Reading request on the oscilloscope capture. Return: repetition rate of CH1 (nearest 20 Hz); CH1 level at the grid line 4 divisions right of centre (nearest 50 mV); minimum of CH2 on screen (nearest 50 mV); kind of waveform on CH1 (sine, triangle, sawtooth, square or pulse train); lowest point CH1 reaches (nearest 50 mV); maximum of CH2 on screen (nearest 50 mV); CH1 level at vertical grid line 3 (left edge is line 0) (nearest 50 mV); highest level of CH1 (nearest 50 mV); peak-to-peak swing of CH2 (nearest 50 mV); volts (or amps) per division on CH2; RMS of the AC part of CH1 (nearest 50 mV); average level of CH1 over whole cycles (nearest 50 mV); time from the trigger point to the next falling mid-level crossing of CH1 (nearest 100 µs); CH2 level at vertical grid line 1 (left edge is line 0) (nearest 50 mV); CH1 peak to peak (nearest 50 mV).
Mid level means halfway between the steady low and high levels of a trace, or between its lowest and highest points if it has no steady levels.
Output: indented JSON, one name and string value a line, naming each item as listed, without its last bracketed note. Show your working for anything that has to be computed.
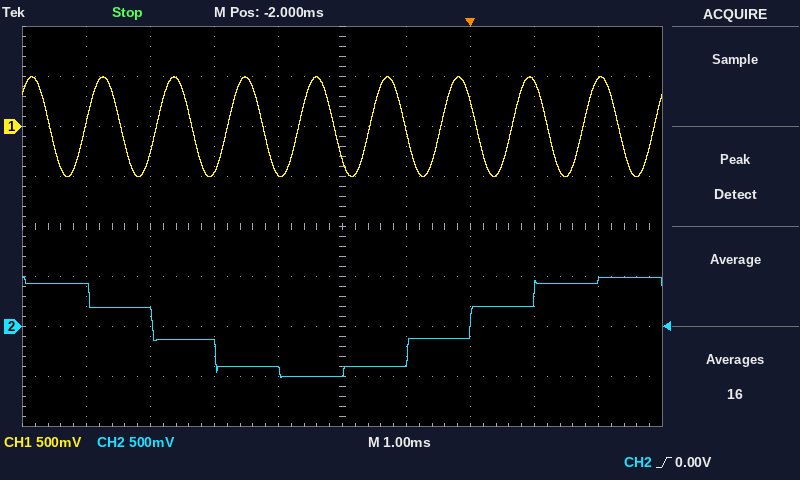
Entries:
{
  "repetition rate of CH1": "900 Hz",
  "CH1 level at the grid line 4 divisions right of centre": "450 mV",
  "minimum of CH2 on screen": "-500 mV",
  "kind of waveform on CH1": "sine",
  "lowest point CH1 reaches": "-500 mV",
  "maximum of CH2 on screen": "500 mV",
  "CH1 level at vertical grid line 3 (left edge is line 0)": "-450 mV",
  "highest level of CH1": "500 mV",
  "peak-to-peak swing of CH2": "500 mV − (-500 mV) = 1.00 V",
  "volts (or amps) per division on CH2": "500 mV",
  "RMS of the AC part of CH1": "1.00 V / (2√2) ≈ 354 mV, so 350 mV to the nearest 50 mV",
  "average level of CH1 over whole cycles": "(500 mV + (-500 mV)) / 2 ≈ 0 mV",
  "time from the trigger point to the next falling mid-level crossing of CH1": "1.2 ms",
  "CH2 level at vertical grid line 1 (left edge is line 0)": "400 mV",
  "CH1 peak to peak": "500 mV − (-500 mV) = 1.00 V"
}
